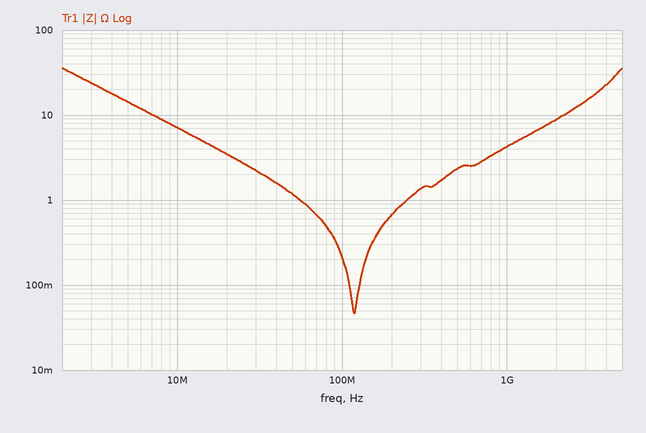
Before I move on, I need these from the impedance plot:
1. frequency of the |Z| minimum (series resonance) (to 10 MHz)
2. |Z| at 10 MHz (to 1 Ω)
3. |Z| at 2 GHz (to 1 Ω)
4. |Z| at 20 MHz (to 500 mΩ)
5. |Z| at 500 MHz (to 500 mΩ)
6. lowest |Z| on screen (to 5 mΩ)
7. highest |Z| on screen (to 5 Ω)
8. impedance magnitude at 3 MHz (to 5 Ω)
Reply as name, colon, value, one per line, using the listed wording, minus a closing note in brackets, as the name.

frequency of the |Z| minimum (series resonance): 120 MHz
|Z| at 10 MHz: 7 Ω
|Z| at 2 GHz: 9 Ω
|Z| at 20 MHz: 3.5 Ω
|Z| at 500 MHz: 2.5 Ω
lowest |Z| on screen: 45 mΩ
highest |Z| on screen: 35 Ω
impedance magnitude at 3 MHz: 25 Ω
